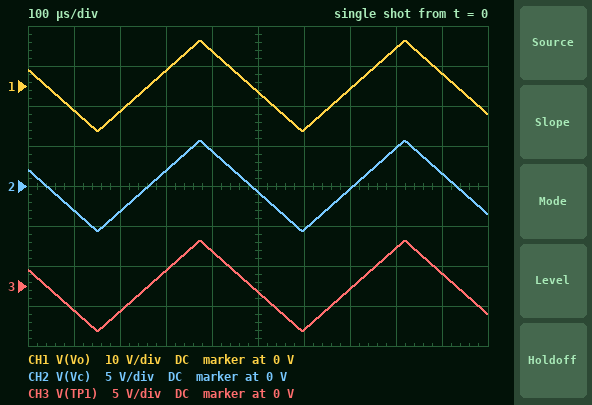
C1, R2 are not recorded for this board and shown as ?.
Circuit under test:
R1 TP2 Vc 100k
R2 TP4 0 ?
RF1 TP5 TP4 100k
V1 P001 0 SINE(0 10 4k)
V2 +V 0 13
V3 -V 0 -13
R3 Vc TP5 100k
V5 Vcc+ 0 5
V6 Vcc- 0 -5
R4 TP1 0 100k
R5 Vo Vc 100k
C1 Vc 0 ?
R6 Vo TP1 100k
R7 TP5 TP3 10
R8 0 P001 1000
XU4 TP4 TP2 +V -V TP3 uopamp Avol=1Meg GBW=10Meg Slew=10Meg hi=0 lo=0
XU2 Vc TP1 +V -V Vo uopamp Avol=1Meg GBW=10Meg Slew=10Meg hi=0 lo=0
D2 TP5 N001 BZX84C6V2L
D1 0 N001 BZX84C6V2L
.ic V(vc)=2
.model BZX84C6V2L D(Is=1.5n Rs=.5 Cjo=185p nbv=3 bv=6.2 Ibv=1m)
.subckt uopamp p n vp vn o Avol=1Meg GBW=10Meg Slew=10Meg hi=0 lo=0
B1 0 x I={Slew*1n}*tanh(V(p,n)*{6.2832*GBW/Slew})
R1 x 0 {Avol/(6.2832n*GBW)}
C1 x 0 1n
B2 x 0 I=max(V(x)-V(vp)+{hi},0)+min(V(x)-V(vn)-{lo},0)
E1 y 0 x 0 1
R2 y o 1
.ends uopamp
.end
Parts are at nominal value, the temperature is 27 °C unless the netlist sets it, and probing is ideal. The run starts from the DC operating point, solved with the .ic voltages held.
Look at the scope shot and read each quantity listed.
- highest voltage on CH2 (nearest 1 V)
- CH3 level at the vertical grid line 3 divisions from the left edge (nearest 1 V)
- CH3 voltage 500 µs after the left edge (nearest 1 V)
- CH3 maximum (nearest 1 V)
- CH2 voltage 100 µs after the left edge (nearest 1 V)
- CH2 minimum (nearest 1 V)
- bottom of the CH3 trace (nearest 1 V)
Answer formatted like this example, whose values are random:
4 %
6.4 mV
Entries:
6 V
2 V
-1 V
6 V
-3 V
-6 V
-6 V
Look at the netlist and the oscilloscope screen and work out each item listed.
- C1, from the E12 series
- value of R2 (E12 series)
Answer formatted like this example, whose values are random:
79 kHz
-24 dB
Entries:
1.5 nF
270 kΩ
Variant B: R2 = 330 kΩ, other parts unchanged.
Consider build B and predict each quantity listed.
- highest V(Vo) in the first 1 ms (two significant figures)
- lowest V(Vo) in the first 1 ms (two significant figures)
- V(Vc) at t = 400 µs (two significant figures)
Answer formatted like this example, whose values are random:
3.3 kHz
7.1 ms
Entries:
12 V
-12 V
5.5 V
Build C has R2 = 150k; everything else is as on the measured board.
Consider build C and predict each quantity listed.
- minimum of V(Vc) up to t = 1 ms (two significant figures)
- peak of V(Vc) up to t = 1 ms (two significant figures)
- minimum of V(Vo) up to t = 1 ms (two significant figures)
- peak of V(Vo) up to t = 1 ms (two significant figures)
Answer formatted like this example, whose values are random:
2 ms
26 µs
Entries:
-4.7 V
4.7 V
-9.3 V
9.3 V
